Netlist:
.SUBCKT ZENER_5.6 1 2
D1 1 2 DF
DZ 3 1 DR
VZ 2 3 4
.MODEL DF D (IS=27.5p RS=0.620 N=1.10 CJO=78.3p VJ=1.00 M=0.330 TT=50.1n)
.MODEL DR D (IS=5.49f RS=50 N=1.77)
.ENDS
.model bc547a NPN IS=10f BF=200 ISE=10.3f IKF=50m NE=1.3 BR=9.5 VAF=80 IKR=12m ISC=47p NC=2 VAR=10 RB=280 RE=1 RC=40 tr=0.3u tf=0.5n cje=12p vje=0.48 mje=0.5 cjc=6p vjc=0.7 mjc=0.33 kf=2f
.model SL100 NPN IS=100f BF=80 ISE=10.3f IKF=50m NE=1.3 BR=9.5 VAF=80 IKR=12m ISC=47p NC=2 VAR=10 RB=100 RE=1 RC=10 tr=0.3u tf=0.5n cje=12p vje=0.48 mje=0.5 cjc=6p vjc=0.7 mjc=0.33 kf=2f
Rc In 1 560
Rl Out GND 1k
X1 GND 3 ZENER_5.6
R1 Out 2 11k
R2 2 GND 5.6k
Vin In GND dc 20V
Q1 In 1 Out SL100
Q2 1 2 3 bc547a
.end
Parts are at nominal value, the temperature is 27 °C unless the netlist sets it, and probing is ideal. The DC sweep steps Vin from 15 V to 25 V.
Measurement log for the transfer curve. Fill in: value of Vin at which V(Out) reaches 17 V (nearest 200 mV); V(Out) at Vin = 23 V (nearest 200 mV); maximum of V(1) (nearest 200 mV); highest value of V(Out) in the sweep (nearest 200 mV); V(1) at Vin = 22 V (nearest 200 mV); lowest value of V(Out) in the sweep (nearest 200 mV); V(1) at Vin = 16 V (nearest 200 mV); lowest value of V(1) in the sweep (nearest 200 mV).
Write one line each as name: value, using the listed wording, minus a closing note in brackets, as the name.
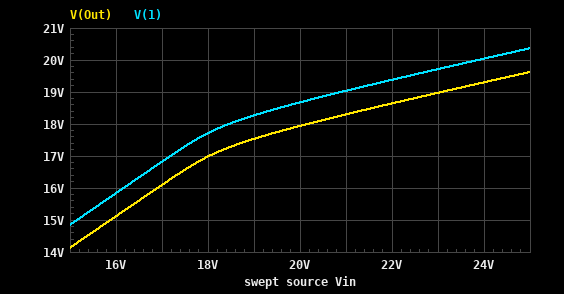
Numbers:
value of Vin at which V(Out) reaches 17 V: 18.0 V
V(Out) at Vin = 23 V: 19.0 V
maximum of V(1): 20.4 V
highest value of V(Out) in the sweep: 19.6 V
V(1) at Vin = 22 V: 19.4 V
lowest value of V(Out) in the sweep: 14.2 V
V(1) at Vin = 16 V: 15.8 V
lowest value of V(1) in the sweep: 14.8 V
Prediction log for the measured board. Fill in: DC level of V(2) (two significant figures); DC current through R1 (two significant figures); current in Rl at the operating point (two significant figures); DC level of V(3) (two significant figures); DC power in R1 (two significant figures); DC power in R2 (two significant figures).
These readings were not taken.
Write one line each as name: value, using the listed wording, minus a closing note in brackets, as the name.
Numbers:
DC level of V(2): 6.0 V
DC current through R1: 1.1 mA
current in Rl at the operating point: 18 mA
DC level of V(3): 5.3 V
DC power in R1: 13 mW
DC power in R2: 6.4 mW
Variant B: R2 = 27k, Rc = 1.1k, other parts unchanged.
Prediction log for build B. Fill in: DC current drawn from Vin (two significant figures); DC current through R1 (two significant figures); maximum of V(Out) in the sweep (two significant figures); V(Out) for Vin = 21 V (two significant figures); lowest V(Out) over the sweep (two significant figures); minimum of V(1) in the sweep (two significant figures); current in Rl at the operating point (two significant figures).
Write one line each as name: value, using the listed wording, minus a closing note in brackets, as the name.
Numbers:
DC current drawn from Vin: 19 mA
DC current through R1: 310 µA
maximum of V(Out) in the sweep: 11 V
V(Out) for Vin = 21 V: 10 V
lowest V(Out) over the sweep: 9.1 V
minimum of V(1) in the sweep: 9.8 V
current in Rl at the operating point: 9.8 mA
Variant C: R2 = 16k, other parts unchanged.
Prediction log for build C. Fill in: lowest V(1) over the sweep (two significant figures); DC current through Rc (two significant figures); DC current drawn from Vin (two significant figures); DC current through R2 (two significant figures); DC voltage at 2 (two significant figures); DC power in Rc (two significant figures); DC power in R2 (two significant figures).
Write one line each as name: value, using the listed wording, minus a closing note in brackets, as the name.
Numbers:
lowest V(1) over the sweep: 12 V
DC current through Rc: 12 mA
DC current drawn from Vin: 25 mA
DC current through R2: 420 µA
DC voltage at 2: 6.7 V
DC power in Rc: 86 mW
DC power in R2: 2.8 mW
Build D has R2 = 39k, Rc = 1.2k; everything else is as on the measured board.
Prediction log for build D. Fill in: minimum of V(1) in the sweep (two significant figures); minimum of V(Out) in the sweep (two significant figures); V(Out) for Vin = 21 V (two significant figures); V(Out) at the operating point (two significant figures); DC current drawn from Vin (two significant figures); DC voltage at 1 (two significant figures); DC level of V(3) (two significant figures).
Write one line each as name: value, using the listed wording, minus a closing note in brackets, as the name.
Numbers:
minimum of V(1) in the sweep: 9.1 V
minimum of V(Out) in the sweep: 8.4 V
V(Out) for Vin = 21 V: 9.2 V
V(Out) at the operating point: 9.0 V
DC current drawn from Vin: 18 mA
DC voltage at 1: 9.7 V
DC level of V(3): 5.7 V
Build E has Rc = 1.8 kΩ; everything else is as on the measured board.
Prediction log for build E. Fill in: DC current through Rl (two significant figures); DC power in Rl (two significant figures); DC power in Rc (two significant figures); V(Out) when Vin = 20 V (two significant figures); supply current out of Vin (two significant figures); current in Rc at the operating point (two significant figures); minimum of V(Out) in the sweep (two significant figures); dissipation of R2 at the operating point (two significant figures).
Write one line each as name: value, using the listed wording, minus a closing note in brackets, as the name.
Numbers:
DC current through Rl: 17 mA
DC power in Rl: 300 mW
DC power in Rc: 1.9 mW
V(Out) when Vin = 20 V: 17 V
supply current out of Vin: 19 mA
current in Rc at the operating point: 1.0 mA
minimum of V(Out) in the sweep: 14 V
dissipation of R2 at the operating point: 6.1 mW
